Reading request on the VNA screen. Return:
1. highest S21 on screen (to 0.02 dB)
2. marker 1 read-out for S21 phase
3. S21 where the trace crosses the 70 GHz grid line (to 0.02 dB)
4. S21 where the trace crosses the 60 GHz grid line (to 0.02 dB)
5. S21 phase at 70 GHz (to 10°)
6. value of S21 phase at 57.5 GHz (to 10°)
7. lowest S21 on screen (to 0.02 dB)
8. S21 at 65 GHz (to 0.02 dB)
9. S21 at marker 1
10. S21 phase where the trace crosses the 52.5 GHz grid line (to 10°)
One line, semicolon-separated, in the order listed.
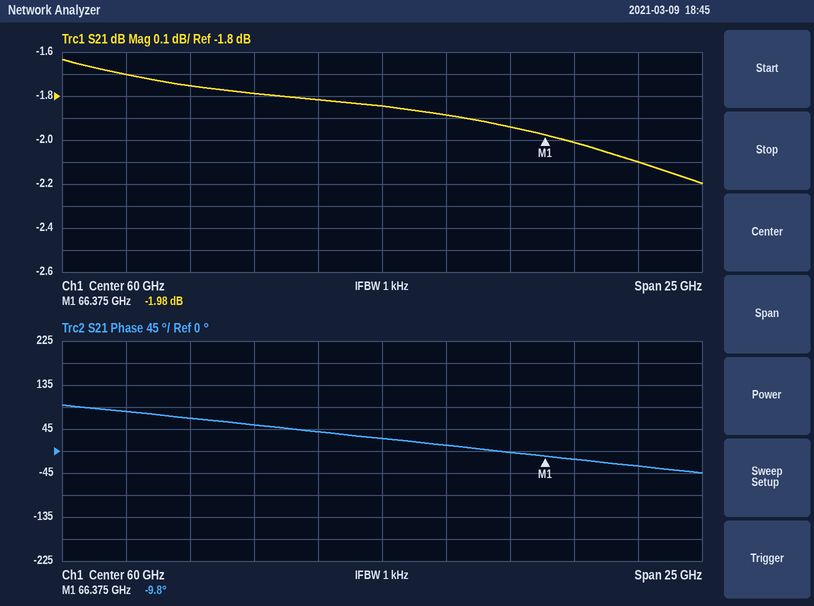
-1.64 dB; -9.8°; -2.10 dB; -1.84 dB; -30°; 40°; -2.20 dB; -1.94 dB; -1.98 dB; 70°
